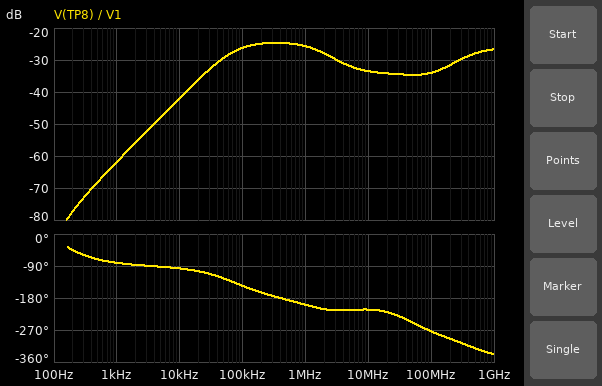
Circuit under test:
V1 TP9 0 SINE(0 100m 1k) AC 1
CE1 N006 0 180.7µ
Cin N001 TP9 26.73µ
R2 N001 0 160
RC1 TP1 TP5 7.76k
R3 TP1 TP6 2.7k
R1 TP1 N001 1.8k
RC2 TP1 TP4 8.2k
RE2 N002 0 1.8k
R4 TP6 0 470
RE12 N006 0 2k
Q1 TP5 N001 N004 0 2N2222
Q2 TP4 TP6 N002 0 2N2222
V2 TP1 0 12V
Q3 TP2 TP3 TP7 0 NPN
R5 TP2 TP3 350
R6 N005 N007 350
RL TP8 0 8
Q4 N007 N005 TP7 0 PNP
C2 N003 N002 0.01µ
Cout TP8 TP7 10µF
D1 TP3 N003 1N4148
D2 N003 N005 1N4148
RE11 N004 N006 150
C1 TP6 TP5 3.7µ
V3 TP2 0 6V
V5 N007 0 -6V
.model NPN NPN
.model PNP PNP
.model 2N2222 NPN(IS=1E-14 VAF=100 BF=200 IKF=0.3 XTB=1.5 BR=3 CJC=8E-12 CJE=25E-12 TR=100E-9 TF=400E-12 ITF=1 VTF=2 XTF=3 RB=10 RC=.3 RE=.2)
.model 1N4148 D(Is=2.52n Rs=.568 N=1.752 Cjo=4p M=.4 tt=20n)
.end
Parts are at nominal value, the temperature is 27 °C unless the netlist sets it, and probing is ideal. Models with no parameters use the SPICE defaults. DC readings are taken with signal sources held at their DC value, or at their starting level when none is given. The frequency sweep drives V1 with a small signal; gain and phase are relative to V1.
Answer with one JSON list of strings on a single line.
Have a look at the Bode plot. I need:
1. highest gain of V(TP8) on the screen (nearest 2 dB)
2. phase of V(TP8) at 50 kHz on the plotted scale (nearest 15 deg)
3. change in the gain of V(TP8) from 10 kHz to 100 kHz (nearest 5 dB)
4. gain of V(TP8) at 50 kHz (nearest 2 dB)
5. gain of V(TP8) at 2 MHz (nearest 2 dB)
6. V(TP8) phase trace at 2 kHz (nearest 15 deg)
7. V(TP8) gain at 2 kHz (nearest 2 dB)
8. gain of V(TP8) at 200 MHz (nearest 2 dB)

["-24 dB", "-120 deg", "15 dB", "-30 dB", "-28 dB", "-90 deg", "-56 dB", "-32 dB"]
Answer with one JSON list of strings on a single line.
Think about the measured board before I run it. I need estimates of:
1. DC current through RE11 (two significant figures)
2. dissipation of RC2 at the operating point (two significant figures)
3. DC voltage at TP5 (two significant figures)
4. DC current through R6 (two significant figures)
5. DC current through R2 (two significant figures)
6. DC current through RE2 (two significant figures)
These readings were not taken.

["170 µA", "3.2 mW", "11 V", "15 mA", "6.1 mA", "630 µA"]
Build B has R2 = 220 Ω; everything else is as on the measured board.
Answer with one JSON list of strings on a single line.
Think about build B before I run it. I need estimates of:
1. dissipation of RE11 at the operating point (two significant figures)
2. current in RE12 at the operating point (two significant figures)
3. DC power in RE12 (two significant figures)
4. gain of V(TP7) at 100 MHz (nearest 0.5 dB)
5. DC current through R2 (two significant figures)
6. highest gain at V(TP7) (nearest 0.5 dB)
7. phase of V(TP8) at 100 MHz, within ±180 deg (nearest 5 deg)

["15 µW", "320 µA", "200 µW", "-32.0 dB", "5.9 mA", "-22.5 dB", "90 deg"]
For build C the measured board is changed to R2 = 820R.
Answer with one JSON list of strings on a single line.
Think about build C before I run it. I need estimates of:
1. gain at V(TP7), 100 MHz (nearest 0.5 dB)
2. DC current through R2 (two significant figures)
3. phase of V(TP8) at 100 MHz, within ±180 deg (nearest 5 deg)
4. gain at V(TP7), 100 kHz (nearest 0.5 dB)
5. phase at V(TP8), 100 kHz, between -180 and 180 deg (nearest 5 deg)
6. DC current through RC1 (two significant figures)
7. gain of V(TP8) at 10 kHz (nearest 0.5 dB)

["-27.0 dB", "4.4 mA", "5 deg", "-38.5 dB", "50 deg", "1.2 mA", "-54.5 dB"]
